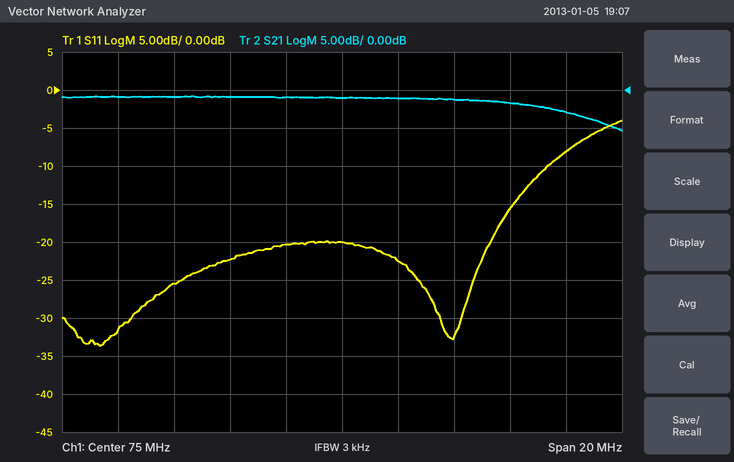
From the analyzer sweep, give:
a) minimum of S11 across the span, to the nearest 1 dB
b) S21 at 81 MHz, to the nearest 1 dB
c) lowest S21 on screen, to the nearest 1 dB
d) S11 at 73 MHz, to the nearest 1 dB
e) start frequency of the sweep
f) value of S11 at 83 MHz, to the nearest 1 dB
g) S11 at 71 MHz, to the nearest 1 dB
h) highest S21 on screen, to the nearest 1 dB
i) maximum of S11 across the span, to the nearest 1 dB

-34 dB
-2 dB
-5 dB
-20 dB
65 MHz
-8 dB
-22 dB
-1 dB
-4 dB
